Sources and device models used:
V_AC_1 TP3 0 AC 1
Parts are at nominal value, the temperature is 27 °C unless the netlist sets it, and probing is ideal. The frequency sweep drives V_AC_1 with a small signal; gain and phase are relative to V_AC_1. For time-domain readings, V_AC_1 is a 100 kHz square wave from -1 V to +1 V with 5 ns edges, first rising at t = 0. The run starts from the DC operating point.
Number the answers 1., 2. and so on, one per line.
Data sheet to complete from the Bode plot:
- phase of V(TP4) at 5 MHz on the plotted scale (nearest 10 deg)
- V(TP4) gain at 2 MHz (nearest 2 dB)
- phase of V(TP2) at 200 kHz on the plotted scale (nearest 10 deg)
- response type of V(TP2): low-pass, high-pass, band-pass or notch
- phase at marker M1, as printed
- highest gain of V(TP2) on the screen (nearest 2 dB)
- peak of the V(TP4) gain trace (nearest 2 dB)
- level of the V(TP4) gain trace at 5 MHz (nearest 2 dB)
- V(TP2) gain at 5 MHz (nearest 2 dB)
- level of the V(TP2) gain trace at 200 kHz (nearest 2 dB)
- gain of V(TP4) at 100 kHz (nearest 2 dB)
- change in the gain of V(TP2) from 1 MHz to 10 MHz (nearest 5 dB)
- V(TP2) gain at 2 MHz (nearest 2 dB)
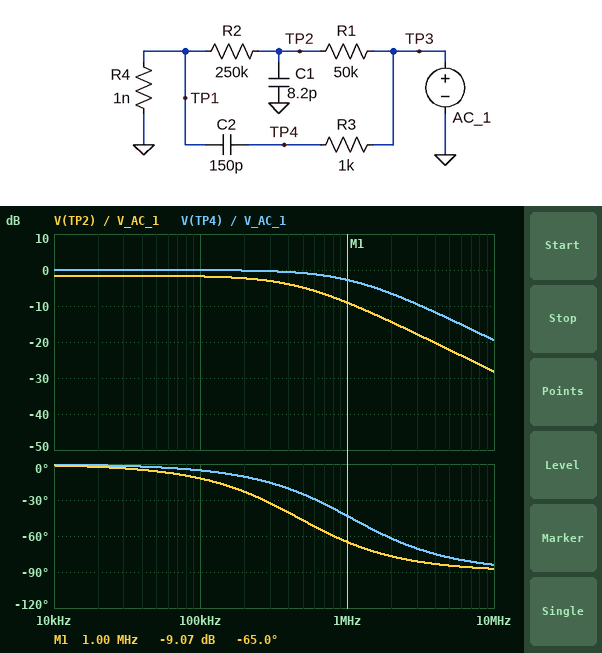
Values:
1. -80 deg
2. -6 dB
3. -20 deg
4. low-pass
5. -65.0 deg
6. -2 dB
7. 0 dB
8. -14 dB
9. -22 dB
10. -2 dB
11. 0 dB
12. -20 dB
13. -14 dB
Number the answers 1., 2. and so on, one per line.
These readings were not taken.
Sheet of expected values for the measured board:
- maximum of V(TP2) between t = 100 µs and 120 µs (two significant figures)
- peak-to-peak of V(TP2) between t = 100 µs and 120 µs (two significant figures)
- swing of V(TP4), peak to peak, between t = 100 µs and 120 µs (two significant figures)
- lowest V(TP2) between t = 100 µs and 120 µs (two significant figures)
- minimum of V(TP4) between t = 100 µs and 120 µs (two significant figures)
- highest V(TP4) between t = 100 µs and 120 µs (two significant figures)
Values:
1. 830 mV
2. 1.7 V
3. 2.0 V
4. -830 mV
5. -1.0 V
6. 1.0 V
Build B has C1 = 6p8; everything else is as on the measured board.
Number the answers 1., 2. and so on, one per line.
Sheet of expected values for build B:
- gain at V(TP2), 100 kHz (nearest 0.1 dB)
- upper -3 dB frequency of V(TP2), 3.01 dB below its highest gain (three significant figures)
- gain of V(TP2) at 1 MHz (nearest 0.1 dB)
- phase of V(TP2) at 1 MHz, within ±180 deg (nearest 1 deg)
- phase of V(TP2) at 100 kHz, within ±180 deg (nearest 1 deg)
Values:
1. -1.7 dB
2. 562 kHz
3. -7.8 dB
4. -61 deg
5. -10 deg
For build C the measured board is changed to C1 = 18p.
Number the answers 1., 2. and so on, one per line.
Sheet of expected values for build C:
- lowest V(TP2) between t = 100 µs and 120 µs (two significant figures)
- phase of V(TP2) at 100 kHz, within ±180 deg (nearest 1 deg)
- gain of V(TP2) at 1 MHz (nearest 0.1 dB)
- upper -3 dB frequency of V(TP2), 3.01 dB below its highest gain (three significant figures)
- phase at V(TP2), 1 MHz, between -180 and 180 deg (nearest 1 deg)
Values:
1. -830 mV
2. -25 deg
3. -15.2 dB
4. 212 kHz
5. -78 deg
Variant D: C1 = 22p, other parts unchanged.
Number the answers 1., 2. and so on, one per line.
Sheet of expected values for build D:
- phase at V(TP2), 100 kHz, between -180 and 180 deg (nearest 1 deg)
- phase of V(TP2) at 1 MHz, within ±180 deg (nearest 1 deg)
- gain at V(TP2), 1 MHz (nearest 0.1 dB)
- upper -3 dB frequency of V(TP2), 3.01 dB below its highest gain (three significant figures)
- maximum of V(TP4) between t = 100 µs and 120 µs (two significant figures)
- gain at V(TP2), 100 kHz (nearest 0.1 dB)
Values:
1. -30 deg
2. -80 deg
3. -16.9 dB
4. 174 kHz
5. 1.0 V
6. -2.8 dB
